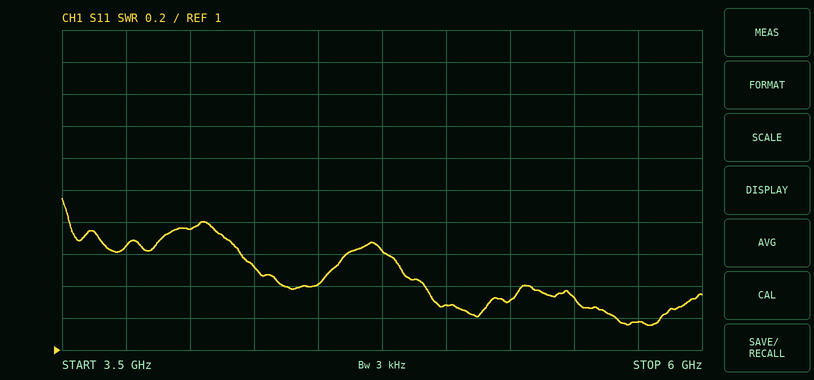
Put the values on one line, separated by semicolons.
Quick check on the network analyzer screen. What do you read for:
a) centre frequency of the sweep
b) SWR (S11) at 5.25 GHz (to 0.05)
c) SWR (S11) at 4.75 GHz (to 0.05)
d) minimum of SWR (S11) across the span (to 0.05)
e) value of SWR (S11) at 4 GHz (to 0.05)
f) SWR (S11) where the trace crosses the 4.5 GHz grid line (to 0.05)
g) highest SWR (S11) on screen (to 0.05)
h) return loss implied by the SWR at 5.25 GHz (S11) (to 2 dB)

4.75 GHz; 1.30; 1.60; 1.15; 1.75; 1.40; 1.95; 18 dB
